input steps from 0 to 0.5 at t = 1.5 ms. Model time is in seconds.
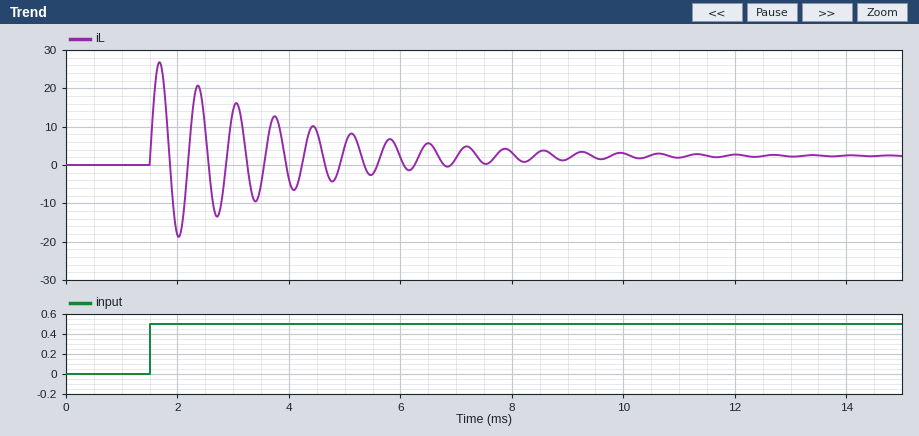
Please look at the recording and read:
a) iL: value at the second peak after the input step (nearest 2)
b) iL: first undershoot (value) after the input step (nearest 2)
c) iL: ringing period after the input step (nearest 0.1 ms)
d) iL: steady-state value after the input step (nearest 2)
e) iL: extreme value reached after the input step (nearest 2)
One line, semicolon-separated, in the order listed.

20; -18; 0.7 ms; 2; 26
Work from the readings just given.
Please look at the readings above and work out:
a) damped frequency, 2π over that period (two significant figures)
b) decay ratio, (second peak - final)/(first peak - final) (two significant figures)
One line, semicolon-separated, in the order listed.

9.0 rad/ms; 0.75
